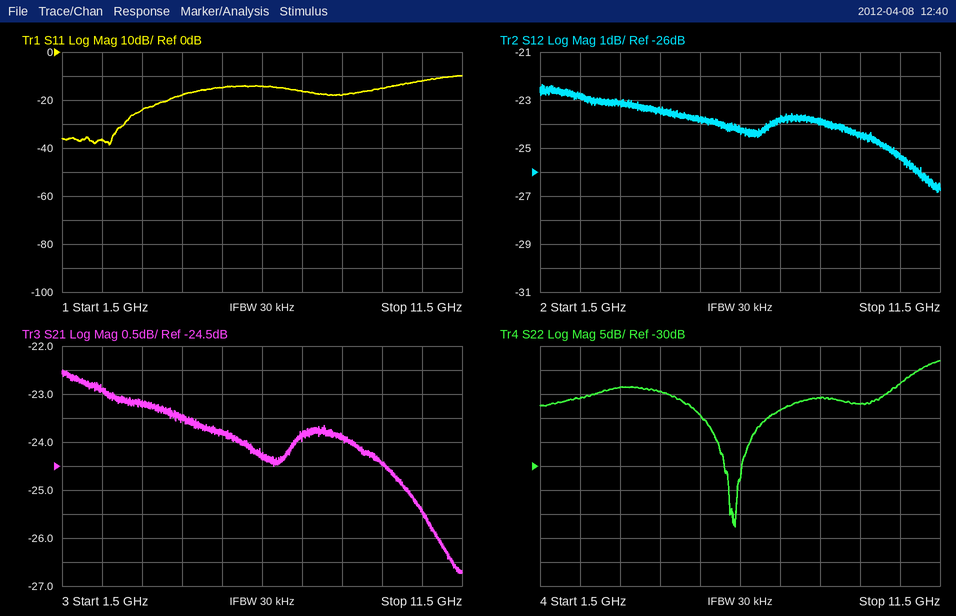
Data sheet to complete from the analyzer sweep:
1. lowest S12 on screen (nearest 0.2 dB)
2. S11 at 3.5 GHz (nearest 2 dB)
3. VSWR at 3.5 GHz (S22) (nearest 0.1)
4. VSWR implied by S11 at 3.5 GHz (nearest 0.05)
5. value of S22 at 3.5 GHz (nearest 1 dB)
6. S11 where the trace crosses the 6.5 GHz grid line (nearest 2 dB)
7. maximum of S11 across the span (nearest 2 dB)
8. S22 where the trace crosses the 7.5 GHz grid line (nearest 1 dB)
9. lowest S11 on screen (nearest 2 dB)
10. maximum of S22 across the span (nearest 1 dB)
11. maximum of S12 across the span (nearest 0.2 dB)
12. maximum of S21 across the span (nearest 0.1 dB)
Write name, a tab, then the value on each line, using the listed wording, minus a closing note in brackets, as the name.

lowest S12 on screen	-26.8 dB
S11 at 3.5 GHz	-24 dB
VSWR at 3.5 GHz (S22)	1.5
VSWR implied by S11 at 3.5 GHz	1.15
value of S22 at 3.5 GHz	-14 dB
S11 where the trace crosses the 6.5 GHz grid line	-14 dB
maximum of S11 across the span	-10 dB
S22 where the trace crosses the 7.5 GHz grid line	-18 dB
lowest S11 on screen	-38 dB
maximum of S22 across the span	-8 dB
maximum of S12 across the span	-22.4 dB
maximum of S21 across the span	-22.5 dB
